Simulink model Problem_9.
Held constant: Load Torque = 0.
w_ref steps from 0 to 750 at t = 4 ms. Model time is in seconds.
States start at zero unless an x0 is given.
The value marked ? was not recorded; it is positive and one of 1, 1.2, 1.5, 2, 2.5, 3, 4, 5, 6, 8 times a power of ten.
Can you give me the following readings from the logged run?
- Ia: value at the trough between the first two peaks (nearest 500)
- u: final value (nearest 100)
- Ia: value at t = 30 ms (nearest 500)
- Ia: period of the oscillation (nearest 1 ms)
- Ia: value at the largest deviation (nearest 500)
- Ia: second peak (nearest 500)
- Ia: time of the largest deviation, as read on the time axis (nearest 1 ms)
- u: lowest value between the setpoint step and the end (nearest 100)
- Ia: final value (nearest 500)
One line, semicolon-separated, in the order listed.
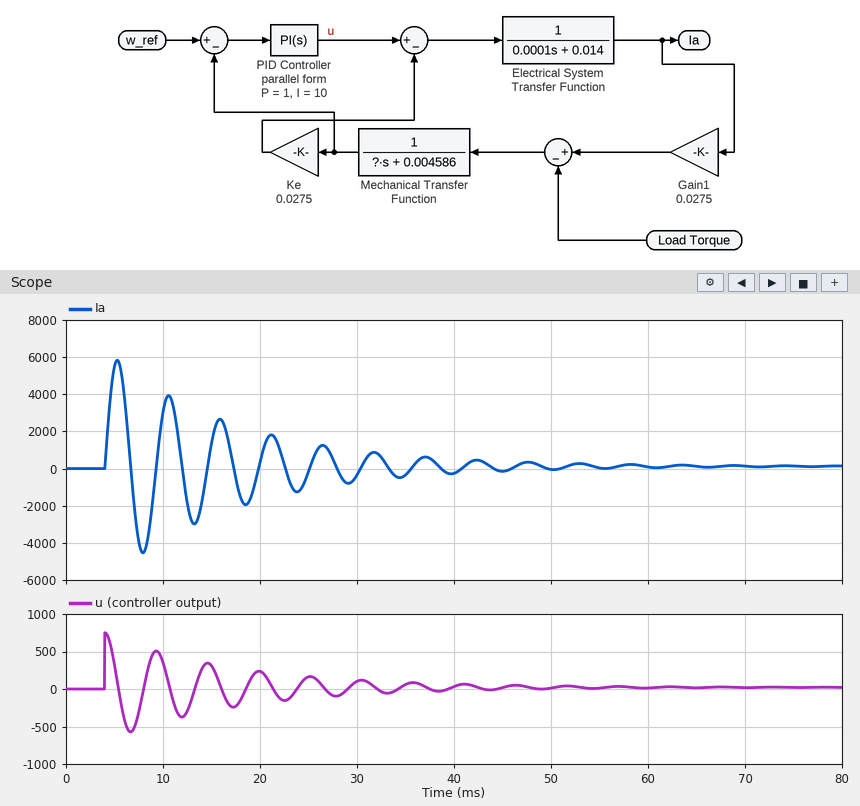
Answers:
-4500; 0; -500; 5 ms; 6000; 4000; 5 ms; -600; 0
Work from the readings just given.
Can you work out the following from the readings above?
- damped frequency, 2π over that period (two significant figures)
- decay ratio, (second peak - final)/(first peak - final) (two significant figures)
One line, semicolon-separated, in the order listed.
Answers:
1.3 rad/ms; 0.67
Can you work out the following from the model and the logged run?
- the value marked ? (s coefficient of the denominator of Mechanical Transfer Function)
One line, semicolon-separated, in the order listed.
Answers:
0.0002
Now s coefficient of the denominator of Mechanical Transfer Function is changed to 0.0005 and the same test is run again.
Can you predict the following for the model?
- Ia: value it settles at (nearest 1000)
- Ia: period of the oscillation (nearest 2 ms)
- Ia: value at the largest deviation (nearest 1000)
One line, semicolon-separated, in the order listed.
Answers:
0; 8 ms; 9000
